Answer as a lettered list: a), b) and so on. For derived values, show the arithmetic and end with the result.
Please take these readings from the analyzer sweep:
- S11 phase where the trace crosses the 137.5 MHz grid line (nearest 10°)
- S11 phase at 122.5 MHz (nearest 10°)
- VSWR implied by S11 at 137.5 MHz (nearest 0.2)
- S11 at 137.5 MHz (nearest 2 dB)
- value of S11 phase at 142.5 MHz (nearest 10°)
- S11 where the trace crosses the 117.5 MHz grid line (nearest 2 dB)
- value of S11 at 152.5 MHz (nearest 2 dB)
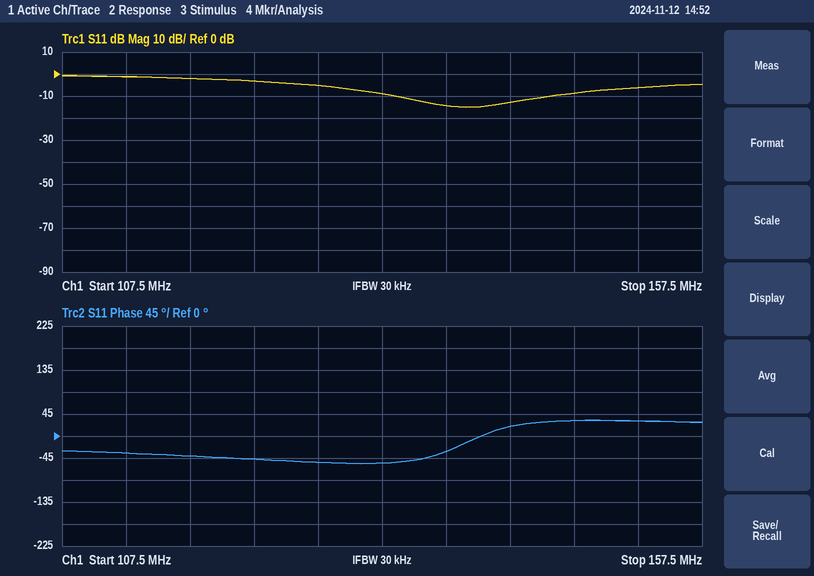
a) -30°
b) -50°
c) |Γ| = 10^(-14/20) = 0.1995; VSWR = (1 + 0.1995)/(1 − 0.1995) ≈ 1.50, so 1.4 to the nearest 0.2
d) -14 dB
e) 20°
f) -2 dB
g) -6 dB
